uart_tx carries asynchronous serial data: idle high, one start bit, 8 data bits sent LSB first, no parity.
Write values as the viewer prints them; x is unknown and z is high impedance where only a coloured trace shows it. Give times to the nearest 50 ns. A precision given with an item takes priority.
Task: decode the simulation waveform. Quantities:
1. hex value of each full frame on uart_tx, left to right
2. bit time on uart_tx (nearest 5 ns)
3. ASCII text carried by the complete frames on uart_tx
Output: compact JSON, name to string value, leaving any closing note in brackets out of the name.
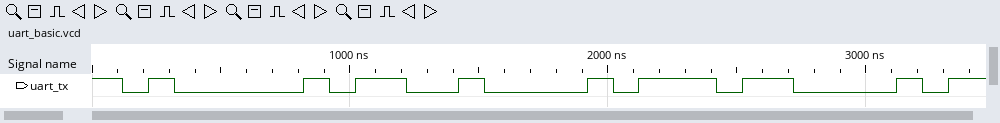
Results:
{"hex value of each full frame on uart_tx, left to right": "41, 42, 43", "bit time on uart_tx": "100 ns", "ASCII text carried by the complete frames on uart_tx": "\"ABC\""}
